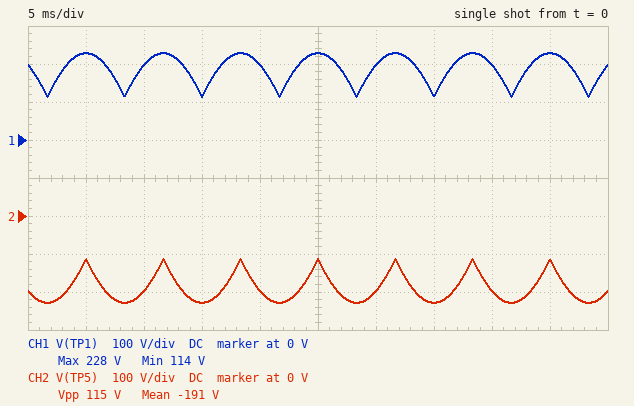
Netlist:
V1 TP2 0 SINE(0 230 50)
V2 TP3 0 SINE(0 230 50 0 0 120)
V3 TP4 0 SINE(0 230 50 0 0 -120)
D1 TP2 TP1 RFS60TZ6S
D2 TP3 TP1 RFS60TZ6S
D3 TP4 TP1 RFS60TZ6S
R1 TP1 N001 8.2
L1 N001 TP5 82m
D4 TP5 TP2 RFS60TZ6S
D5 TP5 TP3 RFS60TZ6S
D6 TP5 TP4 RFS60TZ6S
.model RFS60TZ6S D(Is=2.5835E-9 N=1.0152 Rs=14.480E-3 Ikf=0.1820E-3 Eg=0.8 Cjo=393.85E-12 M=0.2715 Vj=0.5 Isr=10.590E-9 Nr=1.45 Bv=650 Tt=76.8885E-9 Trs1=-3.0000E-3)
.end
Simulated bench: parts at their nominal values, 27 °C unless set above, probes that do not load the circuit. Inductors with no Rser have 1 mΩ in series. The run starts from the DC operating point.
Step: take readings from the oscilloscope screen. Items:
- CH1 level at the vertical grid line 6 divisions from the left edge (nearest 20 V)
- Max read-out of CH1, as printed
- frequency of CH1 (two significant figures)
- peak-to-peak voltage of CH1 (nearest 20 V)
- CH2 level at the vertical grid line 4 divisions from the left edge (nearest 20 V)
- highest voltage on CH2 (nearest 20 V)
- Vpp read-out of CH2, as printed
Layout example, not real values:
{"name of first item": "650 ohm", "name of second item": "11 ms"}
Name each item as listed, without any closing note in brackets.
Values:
{"CH1 level at the vertical grid line 6 divisions from the left edge": "200 V", "Max read-out of CH1, as printed": "228 V", "frequency of CH1": "150 Hz", "peak-to-peak voltage of CH1": "120 V", "CH2 level at the vertical grid line 4 divisions from the left edge": "-200 V", "highest voltage on CH2": "-120 V", "Vpp read-out of CH2, as printed": "115 V"}
